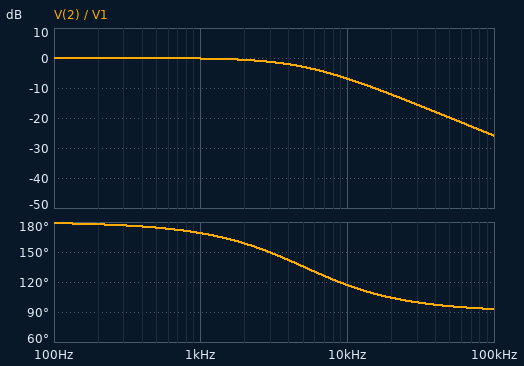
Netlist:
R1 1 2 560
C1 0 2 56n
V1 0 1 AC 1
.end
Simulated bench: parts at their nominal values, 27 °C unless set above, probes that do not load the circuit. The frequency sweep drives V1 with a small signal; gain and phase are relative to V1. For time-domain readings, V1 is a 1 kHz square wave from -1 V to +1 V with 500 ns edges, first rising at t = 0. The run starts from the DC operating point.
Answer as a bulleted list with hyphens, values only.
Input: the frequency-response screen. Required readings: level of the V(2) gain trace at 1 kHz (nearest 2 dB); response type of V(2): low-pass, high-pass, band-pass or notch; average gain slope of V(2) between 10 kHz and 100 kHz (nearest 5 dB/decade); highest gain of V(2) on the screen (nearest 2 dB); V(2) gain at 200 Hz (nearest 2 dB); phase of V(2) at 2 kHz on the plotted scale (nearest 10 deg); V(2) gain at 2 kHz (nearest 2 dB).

- 0 dB
- low-pass
- -20 dB/decade
- 0 dB
- 0 dB
- 160 deg
- 0 dB
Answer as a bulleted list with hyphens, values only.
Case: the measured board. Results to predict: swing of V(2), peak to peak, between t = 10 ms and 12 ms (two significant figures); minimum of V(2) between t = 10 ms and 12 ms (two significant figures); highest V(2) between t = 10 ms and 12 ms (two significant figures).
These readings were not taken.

- 2.0 V
- -1.0 V
- 1.0 V
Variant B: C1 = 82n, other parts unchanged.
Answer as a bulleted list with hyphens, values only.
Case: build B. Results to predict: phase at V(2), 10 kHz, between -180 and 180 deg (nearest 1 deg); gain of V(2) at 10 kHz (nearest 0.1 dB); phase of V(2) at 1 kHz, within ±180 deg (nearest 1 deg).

- 109 deg
- -9.7 dB
- 164 deg
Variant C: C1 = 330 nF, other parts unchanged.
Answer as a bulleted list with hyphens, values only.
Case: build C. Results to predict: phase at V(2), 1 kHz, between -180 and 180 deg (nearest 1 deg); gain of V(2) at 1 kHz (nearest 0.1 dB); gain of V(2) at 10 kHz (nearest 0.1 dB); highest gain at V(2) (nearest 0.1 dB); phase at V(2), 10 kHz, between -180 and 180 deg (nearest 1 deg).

- 131 deg
- -3.7 dB
- -21.3 dB
- 0 dB
- 95 deg
